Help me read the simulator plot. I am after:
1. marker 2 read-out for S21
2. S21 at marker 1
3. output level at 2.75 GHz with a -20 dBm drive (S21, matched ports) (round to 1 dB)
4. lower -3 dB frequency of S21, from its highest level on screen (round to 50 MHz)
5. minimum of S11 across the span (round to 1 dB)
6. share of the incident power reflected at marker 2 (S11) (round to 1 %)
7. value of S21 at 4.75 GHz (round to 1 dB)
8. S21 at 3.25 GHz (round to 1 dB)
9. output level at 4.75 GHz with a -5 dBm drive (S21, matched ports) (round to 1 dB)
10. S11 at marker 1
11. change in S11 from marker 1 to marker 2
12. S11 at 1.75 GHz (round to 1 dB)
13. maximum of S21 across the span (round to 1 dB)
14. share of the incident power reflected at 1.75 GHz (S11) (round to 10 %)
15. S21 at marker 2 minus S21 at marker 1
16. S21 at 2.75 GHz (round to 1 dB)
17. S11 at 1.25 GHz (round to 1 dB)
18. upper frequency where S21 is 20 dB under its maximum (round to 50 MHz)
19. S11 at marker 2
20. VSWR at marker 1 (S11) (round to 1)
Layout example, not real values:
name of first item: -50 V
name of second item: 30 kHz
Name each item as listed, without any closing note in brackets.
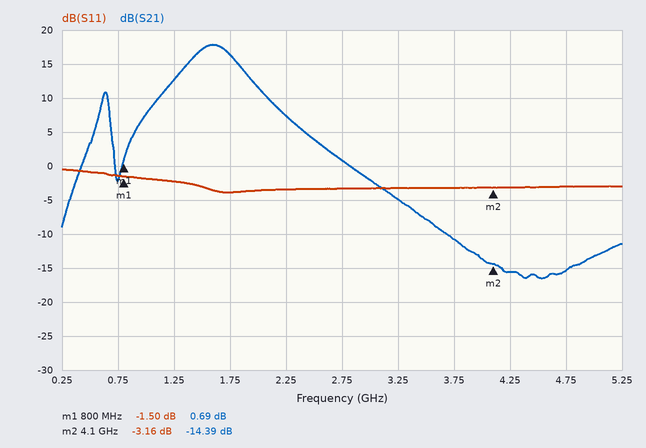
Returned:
marker 2 read-out for S21: -14.39 dB
S21 at marker 1: 0.69 dB
output level at 2.75 GHz with a -20 dBm drive (S21, matched ports): -19 dBm
lower -3 dB frequency of S21, from its highest level on screen: 1.35 GHz
minimum of S11 across the span: -4 dB
share of the incident power reflected at marker 2 (S11): 48 %
value of S21 at 4.75 GHz: -15 dB
S21 at 3.25 GHz: -5 dB
output level at 4.75 GHz with a -5 dBm drive (S21, matched ports): -20 dBm
S11 at marker 1: -1.50 dB
change in S11 from marker 1 to marker 2: -1.66 dB
S11 at 1.75 GHz: -4 dB
maximum of S21 across the span: 18 dB
share of the incident power reflected at 1.75 GHz (S11): 40 %
S21 at marker 2 minus S21 at marker 1: -15.08 dB
S21 at 2.75 GHz: 1 dB
S11 at 1.25 GHz: -2 dB
upper frequency where S21 is 20 dB under its maximum: 3.00 GHz
S11 at marker 2: -3.16 dB
VSWR at marker 1 (S11): 12
